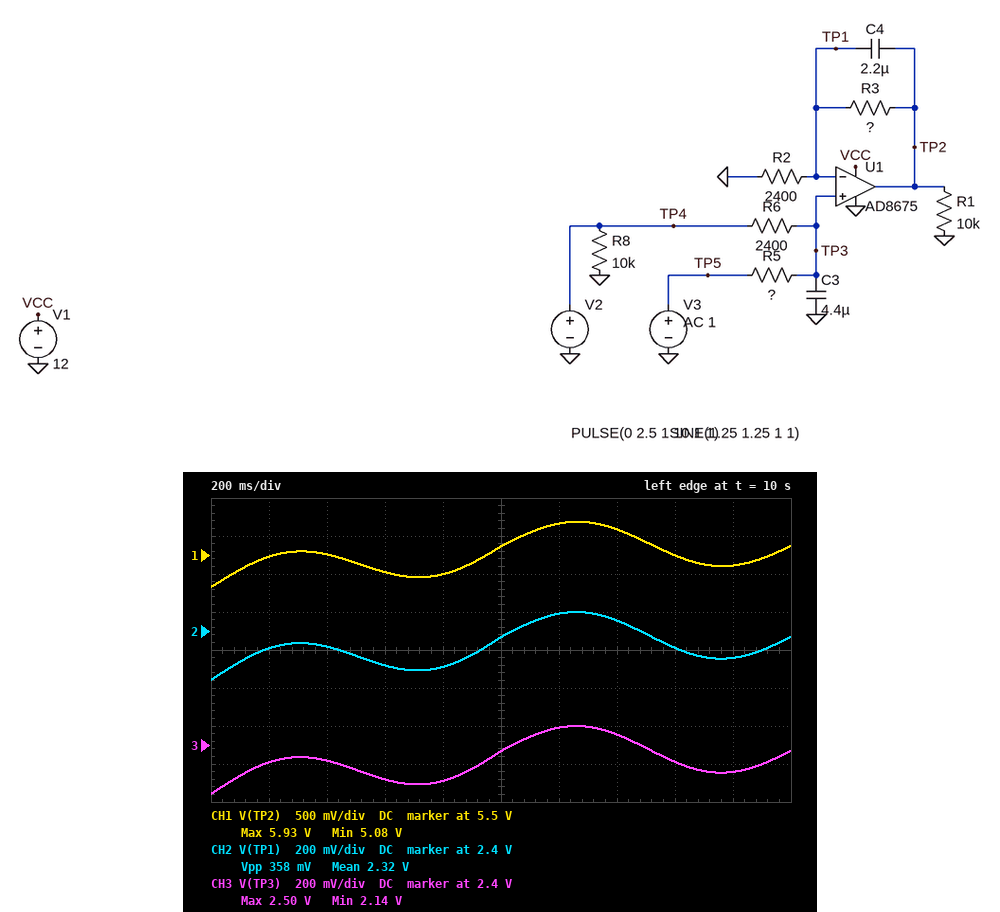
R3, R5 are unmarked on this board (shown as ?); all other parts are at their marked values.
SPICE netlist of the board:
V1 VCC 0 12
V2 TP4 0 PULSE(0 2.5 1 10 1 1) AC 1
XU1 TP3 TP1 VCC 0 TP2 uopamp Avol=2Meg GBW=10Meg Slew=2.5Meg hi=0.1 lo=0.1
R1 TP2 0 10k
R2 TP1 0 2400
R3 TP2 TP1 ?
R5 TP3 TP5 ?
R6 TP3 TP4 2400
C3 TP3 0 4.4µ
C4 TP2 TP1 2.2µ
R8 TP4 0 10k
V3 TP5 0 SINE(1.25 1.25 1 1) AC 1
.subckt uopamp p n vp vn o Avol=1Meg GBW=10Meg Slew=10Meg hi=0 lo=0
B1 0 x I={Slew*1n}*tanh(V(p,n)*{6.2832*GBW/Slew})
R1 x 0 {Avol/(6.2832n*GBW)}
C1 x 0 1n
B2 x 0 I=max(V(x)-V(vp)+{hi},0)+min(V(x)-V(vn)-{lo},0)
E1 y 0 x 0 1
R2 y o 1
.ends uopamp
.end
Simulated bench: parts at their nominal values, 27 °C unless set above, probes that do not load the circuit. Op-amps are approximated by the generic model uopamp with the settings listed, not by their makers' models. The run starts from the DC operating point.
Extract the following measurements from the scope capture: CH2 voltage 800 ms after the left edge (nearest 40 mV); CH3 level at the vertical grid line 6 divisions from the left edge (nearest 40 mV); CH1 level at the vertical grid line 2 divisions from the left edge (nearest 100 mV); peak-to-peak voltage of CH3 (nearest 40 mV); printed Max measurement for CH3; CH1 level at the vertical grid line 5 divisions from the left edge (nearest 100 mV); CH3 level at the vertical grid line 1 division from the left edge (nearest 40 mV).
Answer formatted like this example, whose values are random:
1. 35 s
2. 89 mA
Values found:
1. 2.20 V
2. 2.48 V
3. 5.5 V
4. 360 mV
5. 2.50 V
6. 5.6 V
7. 2.32 V
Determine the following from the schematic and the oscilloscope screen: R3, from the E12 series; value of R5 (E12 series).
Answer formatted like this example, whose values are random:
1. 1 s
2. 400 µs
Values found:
1. 3.3 kΩ
2. 22 kΩ
